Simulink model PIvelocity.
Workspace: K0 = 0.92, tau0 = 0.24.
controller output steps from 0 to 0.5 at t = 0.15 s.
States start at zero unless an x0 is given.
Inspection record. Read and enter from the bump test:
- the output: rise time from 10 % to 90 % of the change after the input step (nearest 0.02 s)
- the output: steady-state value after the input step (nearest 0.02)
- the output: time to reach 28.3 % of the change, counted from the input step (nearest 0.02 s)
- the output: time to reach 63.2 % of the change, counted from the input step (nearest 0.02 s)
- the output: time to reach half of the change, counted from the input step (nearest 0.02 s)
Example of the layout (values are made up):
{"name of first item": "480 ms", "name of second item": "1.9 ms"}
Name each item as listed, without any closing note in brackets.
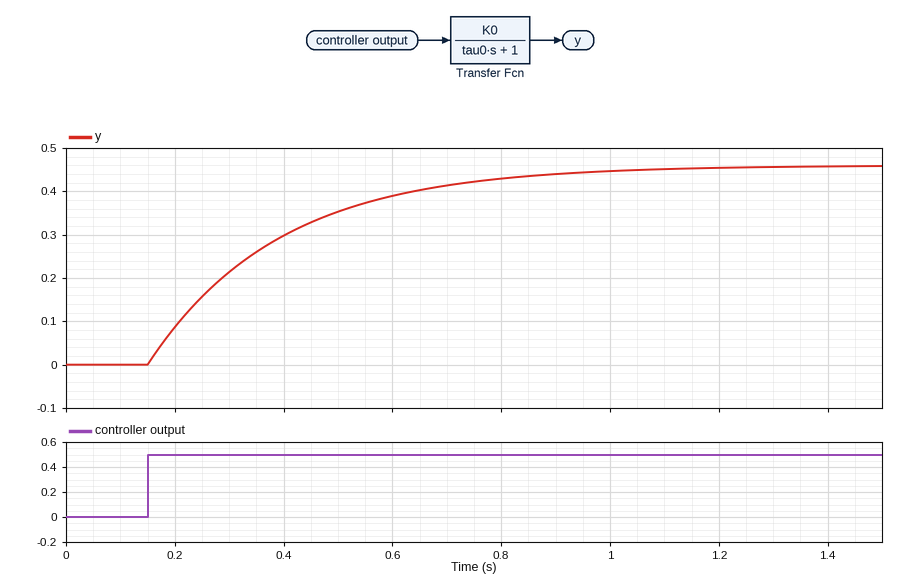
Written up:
{"the output: rise time from 10 % to 90 % of the change after the input step": "0.52 s", "the output: steady-state value after the input step": "0.46", "the output: time to reach 28.3 % of the change, counted from the input step": "0.08 s", "the output: time to reach 63.2 % of the change, counted from the input step": "0.24 s", "the output: time to reach half of the change, counted from the input step": "0.16 s"}
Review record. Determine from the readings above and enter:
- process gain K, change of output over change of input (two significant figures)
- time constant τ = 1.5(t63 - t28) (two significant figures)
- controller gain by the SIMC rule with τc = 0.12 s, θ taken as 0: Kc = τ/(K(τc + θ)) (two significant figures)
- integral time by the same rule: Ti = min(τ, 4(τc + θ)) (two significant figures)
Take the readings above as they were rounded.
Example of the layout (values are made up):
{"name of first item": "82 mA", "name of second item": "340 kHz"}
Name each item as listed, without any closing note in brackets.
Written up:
{"process gain K, change of output over change of input": "0.92", "time constant τ = 1.5(t63 - t28)": "0.24 s", "controller gain by the SIMC rule with τc = 0.12 s, θ taken as 0: Kc = τ/(K(τc + θ))": "2.2", "integral time by the same rule: Ti = min(τ, 4(τc + θ))": "0.24 s"}
